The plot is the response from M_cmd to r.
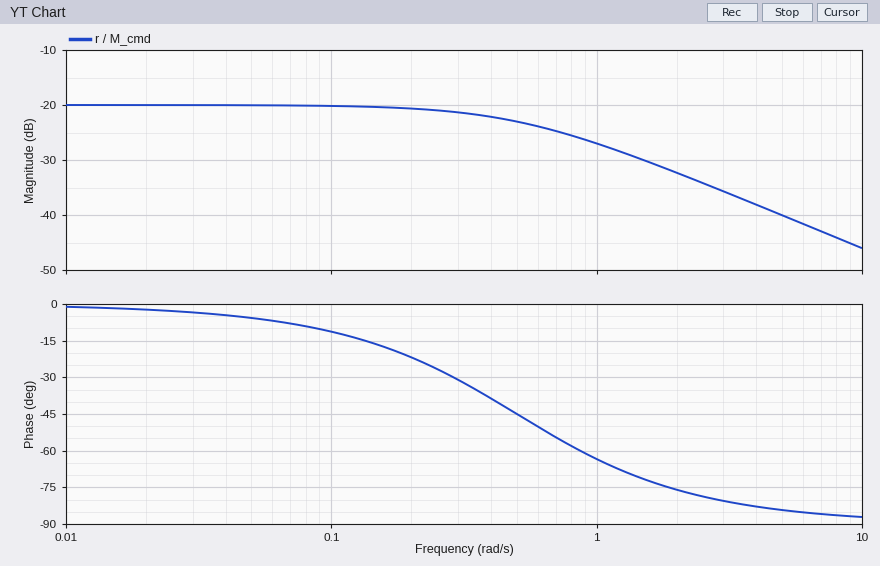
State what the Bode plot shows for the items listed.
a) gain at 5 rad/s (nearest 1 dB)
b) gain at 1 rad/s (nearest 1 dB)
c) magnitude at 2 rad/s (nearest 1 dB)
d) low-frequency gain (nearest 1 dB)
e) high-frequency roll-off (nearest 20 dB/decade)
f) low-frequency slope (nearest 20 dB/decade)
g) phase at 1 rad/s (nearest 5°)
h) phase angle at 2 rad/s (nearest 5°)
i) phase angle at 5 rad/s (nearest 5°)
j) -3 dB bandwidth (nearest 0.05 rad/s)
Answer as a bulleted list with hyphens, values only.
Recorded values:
- -40 dB
- -27 dB
- -32 dB
- -20 dB
- -20 dB/decade
- 0 dB/decade
- -65°
- -75°
- -85°
- 0.50 rad/s
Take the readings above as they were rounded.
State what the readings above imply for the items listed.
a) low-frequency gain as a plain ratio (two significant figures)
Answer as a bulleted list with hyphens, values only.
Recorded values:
- 0.10
